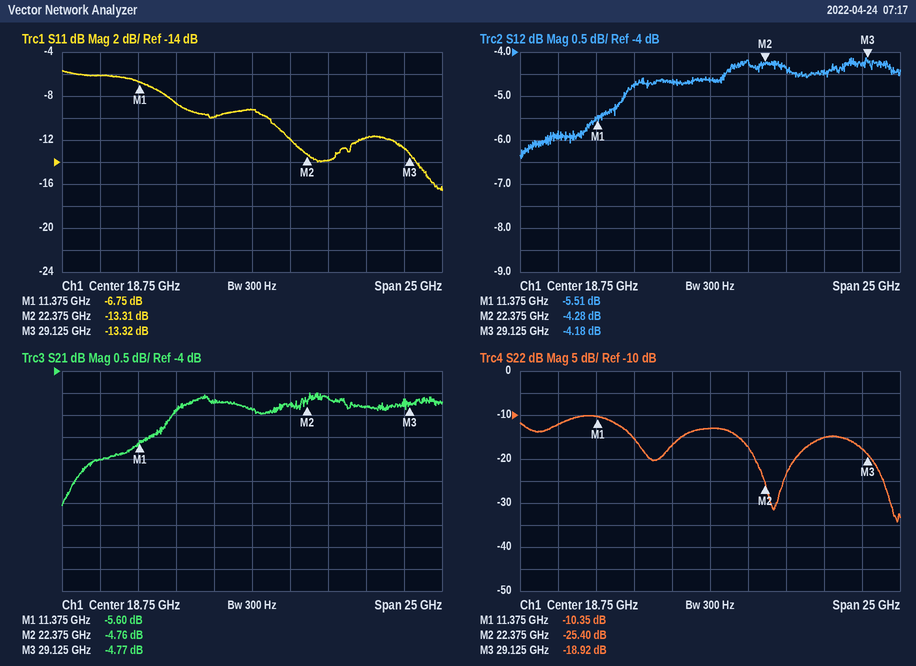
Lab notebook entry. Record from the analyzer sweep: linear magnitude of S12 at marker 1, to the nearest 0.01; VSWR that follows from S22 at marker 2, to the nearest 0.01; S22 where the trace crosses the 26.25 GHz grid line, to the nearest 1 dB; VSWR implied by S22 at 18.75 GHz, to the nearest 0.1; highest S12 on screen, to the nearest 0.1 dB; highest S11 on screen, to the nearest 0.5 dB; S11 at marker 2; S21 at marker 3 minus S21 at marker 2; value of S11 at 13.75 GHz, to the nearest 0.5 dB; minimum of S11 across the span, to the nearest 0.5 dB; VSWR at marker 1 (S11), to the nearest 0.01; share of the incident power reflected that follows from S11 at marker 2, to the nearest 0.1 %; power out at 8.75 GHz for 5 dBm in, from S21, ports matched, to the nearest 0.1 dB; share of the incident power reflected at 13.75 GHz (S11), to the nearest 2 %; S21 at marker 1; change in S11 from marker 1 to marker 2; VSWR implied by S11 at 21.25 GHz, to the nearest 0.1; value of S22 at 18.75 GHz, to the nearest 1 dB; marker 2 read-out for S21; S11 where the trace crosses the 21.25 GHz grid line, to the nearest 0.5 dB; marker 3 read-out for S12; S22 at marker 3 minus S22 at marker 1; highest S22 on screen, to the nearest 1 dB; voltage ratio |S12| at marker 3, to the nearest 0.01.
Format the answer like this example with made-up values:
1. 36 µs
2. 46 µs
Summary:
1. 0.53
2. 1.11
3. -15 dB
4. 1.6
5. -4.1 dB
6. -5.5 dB
7. -13.31 dB
8. -0.01 dB
9. -8.5 dB
10. -16.5 dB
11. 2.70
12. 4.7 %
13. -1.0 dBm
14. 14 %
15. -5.60 dB
16. -6.56 dB
17. 1.7
18. -13 dB
19. -4.76 dB
20. -12.0 dB
21. -4.18 dB
22. -8.57 dB
23. -10 dB
24. 0.62
